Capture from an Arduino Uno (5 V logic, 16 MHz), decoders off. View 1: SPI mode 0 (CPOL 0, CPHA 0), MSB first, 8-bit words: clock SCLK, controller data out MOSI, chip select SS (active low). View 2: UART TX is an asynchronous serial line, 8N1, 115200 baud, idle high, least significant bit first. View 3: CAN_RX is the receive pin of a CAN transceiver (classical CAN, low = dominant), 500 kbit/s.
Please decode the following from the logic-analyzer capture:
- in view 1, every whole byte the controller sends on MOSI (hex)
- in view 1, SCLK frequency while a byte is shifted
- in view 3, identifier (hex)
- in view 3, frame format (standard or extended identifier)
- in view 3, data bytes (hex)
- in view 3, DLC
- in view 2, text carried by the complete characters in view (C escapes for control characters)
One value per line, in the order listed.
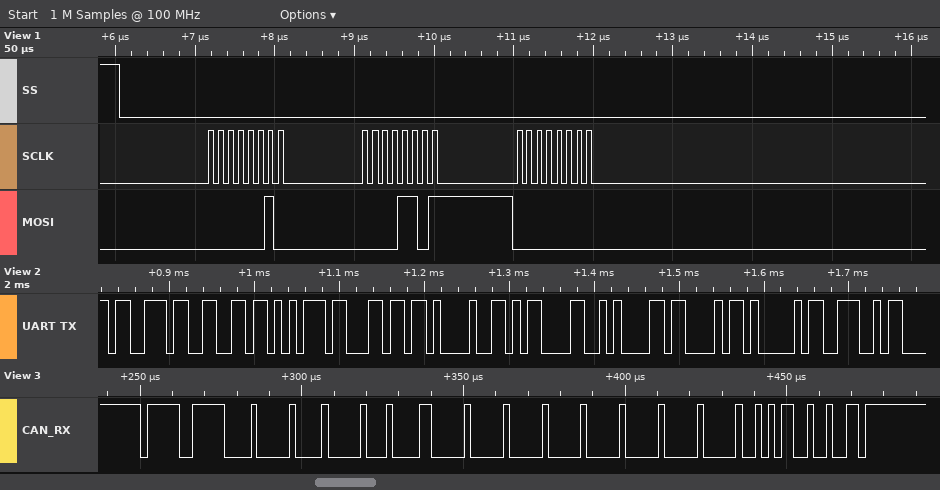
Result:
0x02 0x0D 0x00
8 MHz
0x7DF
standard
02 01 0C 00 00 00 00 00
8
"sful!\r\nCAN"
